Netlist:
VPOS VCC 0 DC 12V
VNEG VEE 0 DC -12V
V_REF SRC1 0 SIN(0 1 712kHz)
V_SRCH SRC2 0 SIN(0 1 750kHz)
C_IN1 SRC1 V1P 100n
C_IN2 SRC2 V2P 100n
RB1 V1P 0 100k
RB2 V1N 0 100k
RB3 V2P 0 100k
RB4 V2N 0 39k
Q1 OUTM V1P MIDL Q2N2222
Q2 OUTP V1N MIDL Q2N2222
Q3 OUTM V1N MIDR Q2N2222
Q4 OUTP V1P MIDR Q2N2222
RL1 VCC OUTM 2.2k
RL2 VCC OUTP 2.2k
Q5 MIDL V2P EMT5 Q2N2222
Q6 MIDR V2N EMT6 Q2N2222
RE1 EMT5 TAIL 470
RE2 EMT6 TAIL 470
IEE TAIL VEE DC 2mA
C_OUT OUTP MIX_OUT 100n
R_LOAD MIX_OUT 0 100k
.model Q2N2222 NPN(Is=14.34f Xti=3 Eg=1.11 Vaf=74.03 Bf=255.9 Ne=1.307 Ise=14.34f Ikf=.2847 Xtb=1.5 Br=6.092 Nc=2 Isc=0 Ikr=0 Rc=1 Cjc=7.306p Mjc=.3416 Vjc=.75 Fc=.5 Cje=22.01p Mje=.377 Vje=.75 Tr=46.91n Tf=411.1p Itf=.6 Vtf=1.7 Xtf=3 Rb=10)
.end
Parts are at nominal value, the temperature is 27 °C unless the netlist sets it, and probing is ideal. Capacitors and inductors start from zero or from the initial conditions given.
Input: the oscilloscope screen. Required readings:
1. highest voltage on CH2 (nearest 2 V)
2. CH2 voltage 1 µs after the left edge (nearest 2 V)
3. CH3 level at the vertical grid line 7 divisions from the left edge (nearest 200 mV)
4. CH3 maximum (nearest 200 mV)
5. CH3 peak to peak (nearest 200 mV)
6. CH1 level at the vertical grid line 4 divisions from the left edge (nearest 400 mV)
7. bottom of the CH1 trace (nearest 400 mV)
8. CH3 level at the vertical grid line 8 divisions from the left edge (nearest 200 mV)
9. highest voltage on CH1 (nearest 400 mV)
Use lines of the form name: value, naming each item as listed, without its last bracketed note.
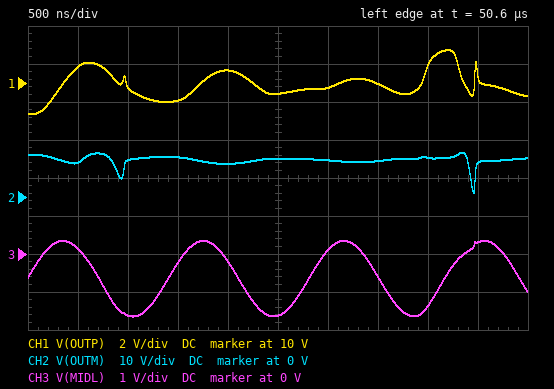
highest voltage on CH2: 12 V
CH2 voltage 1 µs after the left edge: 10 V
CH3 level at the vertical grid line 7 divisions from the left edge: -600 mV
CH3 maximum: 400 mV
CH3 peak to peak: 2.0 V
CH1 level at the vertical grid line 4 divisions from the left edge: 10.8 V
bottom of the CH1 trace: 8.4 V
CH3 level at the vertical grid line 8 divisions from the left edge: -1.4 V
highest voltage on CH1: 11.6 V
